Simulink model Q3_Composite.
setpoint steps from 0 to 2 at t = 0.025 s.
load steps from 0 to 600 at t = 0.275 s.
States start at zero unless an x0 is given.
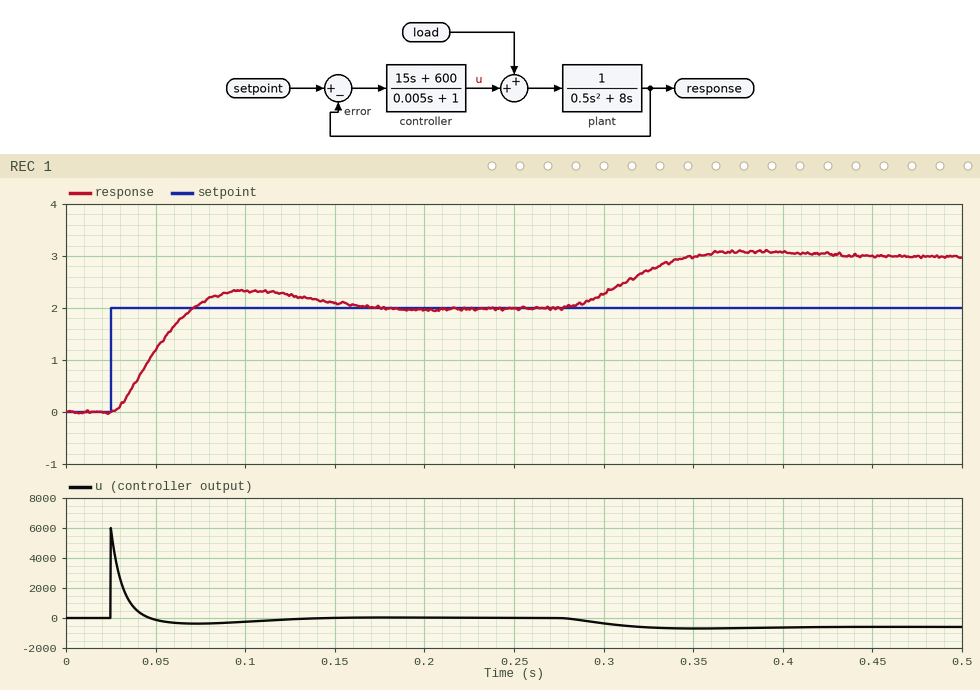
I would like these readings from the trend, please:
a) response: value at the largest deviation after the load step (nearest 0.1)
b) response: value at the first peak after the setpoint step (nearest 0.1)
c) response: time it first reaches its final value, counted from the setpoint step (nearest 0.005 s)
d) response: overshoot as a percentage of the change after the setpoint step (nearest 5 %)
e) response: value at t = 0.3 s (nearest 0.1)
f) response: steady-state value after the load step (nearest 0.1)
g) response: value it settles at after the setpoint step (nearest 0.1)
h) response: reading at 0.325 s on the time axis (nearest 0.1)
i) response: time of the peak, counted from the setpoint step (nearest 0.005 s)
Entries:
3.1
2.3
0.045 s
15 %
2.3
3.0
2.0
2.7
0.075 s
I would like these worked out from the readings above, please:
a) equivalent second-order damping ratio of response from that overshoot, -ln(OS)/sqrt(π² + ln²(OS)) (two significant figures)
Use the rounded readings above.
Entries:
0.52
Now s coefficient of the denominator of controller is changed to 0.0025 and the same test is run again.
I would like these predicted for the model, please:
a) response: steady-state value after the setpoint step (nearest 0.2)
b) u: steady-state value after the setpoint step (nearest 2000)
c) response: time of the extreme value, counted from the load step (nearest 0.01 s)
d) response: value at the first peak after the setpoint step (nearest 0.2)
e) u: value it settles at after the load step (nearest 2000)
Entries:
2.0
0
0.11 s
2.2
0
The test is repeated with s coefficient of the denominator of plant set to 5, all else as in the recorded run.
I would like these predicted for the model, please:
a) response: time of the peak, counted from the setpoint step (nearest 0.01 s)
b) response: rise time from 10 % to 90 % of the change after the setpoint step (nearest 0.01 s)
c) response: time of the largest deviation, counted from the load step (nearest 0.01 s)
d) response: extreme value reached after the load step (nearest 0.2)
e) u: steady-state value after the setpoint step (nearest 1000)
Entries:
0.07 s
0.03 s
0.10 s
3.2
0
